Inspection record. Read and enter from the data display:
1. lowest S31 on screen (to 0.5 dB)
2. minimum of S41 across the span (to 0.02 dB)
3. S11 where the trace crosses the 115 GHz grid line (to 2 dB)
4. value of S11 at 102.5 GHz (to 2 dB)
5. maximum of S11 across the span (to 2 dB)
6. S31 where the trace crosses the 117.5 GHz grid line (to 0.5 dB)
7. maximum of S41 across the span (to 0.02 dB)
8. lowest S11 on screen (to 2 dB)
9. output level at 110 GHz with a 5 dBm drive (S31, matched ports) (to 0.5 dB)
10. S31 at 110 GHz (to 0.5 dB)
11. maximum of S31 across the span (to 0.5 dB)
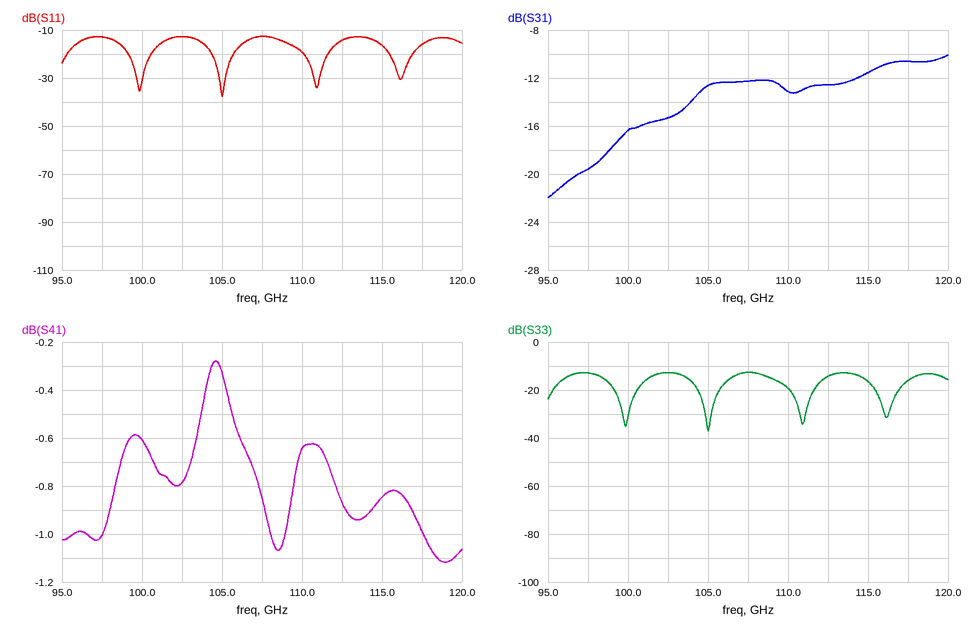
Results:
-22.0 dB
-1.12 dB
-16 dB
-12 dB
-12 dB
-10.5 dB
-0.28 dB
-38 dB
-8.0 dBm
-13.0 dB
-10.0 dB
